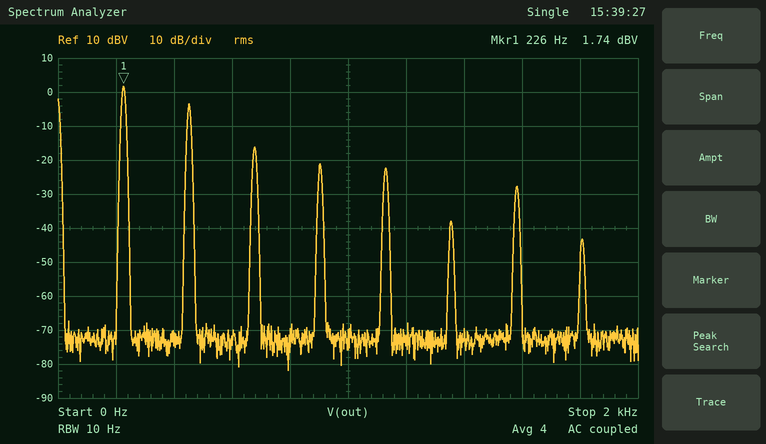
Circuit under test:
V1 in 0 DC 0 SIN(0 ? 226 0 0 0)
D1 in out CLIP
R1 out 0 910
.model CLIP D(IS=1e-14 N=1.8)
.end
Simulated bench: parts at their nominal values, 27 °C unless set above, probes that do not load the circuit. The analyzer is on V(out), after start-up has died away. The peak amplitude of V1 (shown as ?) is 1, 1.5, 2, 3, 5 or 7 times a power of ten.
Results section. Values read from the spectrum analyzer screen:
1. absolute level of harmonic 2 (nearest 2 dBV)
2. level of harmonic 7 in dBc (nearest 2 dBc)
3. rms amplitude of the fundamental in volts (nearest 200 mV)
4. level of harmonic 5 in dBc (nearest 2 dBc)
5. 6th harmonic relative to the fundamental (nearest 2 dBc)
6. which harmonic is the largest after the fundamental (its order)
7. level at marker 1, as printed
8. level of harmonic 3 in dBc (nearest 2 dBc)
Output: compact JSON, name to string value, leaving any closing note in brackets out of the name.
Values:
{"absolute level of harmonic 2": "-4 dBV", "level of harmonic 7 in dBc": "-30 dBc", "rms amplitude of the fundamental in volts": "1.2 V", "level of harmonic 5 in dBc": "-24 dBc", "6th harmonic relative to the fundamental": "-40 dBc", "which harmonic is the largest after the fundamental": "2", "level at marker 1, as printed": "1.74 dBV", "level of harmonic 3 in dBc": "-18 dBc"}
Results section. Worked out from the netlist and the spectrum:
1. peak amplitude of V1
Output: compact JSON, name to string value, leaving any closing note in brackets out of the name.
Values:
{"peak amplitude of V1": "5 V"}
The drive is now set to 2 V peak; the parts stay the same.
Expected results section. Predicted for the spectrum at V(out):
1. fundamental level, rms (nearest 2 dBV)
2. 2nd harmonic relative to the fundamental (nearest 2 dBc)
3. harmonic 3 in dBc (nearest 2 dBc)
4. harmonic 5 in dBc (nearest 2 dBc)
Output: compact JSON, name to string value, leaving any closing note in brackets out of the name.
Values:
{"fundamental level, rms": "-14 dBV", "2nd harmonic relative to the fundamental": "-2 dBc", "harmonic 3 in dBc": "-8 dBc", "harmonic 5 in dBc": "-28 dBc"}
